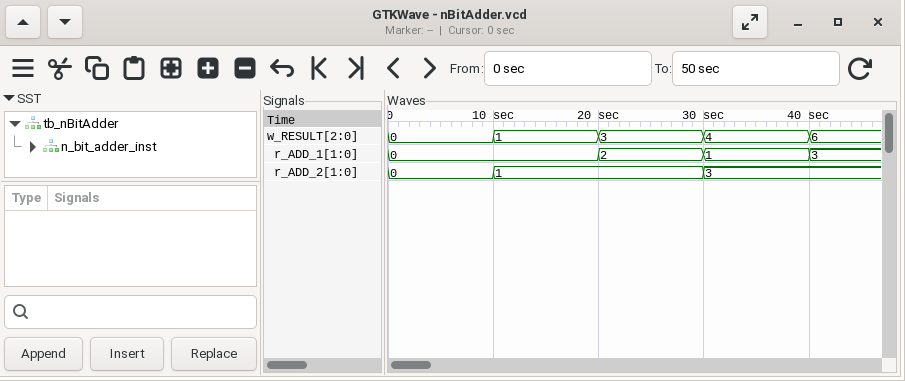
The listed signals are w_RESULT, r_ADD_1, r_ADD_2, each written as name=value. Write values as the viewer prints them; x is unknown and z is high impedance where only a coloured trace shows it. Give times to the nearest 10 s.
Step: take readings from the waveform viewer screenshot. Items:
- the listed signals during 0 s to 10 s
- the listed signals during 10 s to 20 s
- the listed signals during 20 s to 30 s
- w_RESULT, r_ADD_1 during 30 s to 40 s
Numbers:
w_RESULT=0, r_ADD_1=0, r_ADD_2=0
w_RESULT=1, r_ADD_1=0, r_ADD_2=1
w_RESULT=3, r_ADD_1=2, r_ADD_2=1
w_RESULT=4, r_ADD_1=1
